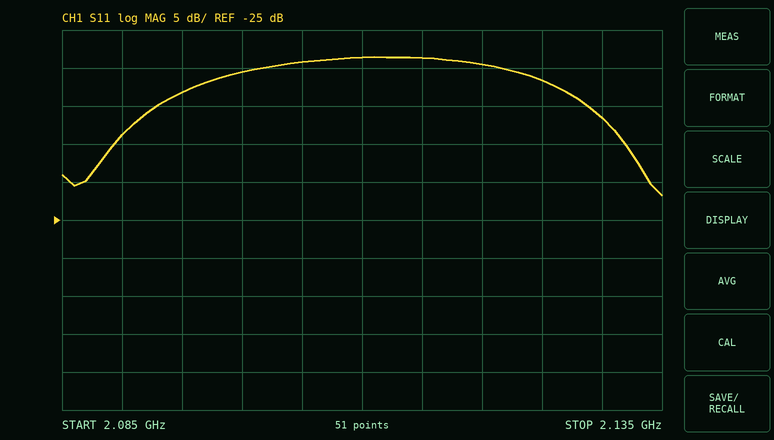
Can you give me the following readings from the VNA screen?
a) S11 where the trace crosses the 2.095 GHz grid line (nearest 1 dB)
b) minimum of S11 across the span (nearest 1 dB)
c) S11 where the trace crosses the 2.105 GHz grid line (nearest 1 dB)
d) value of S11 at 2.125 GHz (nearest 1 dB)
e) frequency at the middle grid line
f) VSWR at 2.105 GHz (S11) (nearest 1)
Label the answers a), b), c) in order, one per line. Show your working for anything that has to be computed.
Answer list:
a) -8 dB
b) -22 dB
c) -4 dB
d) -7 dB
e) 2.11 GHz
f) |Γ| = 10^(-4/20) = 0.6310; VSWR = (1 + 0.6310)/(1 − 0.6310) ≈ 4
